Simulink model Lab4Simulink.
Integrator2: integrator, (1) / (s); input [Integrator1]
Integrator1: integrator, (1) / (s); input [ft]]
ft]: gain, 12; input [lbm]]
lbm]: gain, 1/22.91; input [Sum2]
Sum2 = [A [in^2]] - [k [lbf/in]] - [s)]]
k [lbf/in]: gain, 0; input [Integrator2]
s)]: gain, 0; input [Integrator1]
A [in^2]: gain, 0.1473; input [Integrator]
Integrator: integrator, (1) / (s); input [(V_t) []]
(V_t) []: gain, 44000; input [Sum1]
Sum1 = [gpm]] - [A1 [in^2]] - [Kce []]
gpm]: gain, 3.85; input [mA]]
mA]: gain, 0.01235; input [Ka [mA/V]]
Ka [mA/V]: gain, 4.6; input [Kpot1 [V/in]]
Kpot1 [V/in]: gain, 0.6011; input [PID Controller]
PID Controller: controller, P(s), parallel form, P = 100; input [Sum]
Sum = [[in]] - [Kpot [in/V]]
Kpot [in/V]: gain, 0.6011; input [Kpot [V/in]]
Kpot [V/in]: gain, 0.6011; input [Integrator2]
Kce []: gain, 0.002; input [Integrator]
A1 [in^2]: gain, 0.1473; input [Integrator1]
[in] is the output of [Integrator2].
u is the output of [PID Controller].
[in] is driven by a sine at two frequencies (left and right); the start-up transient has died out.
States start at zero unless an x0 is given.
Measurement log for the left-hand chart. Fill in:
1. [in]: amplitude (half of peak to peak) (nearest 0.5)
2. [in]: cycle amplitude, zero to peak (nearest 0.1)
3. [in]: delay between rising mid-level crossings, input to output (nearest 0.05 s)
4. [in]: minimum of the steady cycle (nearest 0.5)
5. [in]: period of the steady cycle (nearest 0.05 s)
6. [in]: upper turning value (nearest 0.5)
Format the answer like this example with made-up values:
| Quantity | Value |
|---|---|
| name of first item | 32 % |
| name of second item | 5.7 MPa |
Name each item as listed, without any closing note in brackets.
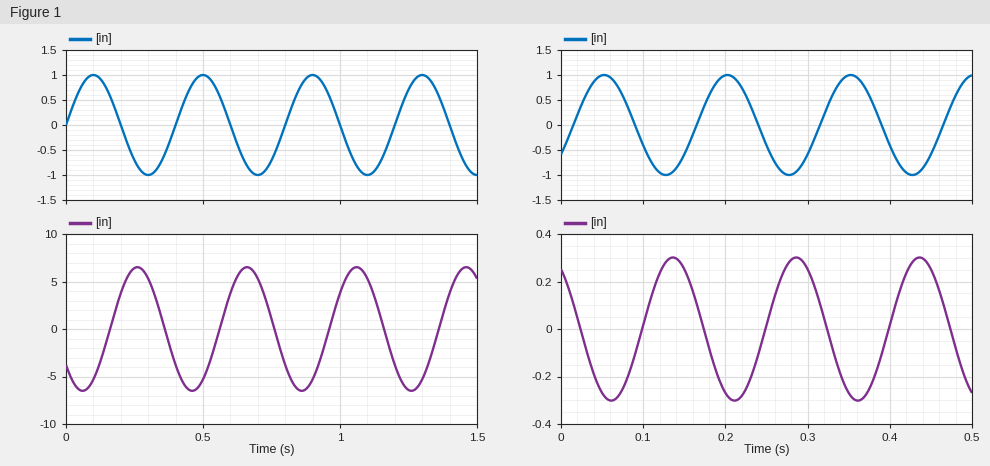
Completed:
| Quantity | Value |
|---|---|
| [in]: amplitude (half of peak to peak) | 6.5 |
| [in]: cycle amplitude, zero to peak | 1.0 |
| [in]: delay between rising mid-level crossings, input to output | 0.15 s |
| [in]: minimum of the steady cycle | -6.5 |
| [in]: period of the steady cycle | 0.40 s |
| [in]: upper turning value | 6.5 |
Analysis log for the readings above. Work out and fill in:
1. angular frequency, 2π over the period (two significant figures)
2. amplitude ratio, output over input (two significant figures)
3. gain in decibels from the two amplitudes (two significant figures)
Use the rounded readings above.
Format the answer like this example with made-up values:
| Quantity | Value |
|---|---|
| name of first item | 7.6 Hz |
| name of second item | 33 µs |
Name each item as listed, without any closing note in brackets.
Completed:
| Quantity | Value |
|---|---|
| angular frequency, 2π over the period | 16 rad/s |
| amplitude ratio, output over input | 6.5 |
| gain in decibels from the two amplitudes | 16 dB |
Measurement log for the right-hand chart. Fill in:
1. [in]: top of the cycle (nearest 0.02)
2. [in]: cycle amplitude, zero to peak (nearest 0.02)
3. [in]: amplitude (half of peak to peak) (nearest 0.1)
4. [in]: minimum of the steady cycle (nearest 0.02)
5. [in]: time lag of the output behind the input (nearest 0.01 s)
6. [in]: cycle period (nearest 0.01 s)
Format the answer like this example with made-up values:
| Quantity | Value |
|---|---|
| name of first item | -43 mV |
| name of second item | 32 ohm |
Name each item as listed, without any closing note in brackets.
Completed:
| Quantity | Value |
|---|---|
| [in]: top of the cycle | 0.30 |
| [in]: cycle amplitude, zero to peak | 0.30 |
| [in]: amplitude (half of peak to peak) | 1.0 |
| [in]: minimum of the steady cycle | -0.30 |
| [in]: time lag of the output behind the input | 0.08 s |
| [in]: cycle period | 0.15 s |
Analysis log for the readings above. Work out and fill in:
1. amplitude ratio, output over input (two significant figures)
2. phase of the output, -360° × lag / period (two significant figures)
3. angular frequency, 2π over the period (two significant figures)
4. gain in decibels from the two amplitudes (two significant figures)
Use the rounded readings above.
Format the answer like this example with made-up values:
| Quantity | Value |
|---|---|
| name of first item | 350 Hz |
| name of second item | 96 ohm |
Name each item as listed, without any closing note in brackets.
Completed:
| Quantity | Value |
|---|---|
| amplitude ratio, output over input | 0.30 |
| phase of the output, -360° × lag / period | -190° |
| angular frequency, 2π over the period | 42 rad/s |
| gain in decibels from the two amplitudes | -10 dB |
